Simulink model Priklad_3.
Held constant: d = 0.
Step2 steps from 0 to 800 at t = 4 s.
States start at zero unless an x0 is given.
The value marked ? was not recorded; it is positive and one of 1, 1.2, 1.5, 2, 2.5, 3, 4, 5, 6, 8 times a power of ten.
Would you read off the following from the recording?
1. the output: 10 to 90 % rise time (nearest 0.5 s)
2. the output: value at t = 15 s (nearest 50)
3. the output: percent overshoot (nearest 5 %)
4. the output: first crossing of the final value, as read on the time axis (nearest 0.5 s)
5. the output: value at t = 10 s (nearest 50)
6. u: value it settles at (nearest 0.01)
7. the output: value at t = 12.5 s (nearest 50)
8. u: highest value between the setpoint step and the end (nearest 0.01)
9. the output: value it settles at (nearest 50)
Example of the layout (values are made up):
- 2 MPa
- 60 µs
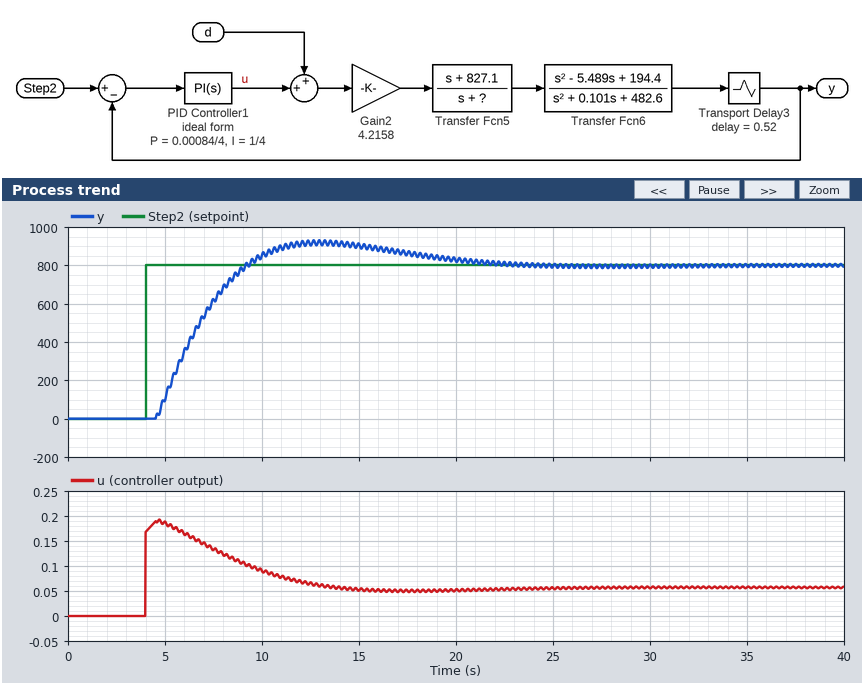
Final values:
- 3.5 s
- 900
- 15 %
- 9.0 s
- 850
- 0.06
- 900
- 0.19
- 800
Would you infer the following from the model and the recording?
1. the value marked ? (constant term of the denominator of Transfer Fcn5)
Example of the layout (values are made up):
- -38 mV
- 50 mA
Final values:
- 0.1
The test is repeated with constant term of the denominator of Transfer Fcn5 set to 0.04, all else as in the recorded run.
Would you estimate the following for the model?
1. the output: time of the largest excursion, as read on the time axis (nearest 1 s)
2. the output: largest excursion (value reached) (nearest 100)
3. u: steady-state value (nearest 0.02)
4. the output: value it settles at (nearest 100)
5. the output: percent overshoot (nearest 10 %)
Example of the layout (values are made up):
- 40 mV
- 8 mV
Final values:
- 12 s
- 1000
- 0.02
- 800
- 30 %
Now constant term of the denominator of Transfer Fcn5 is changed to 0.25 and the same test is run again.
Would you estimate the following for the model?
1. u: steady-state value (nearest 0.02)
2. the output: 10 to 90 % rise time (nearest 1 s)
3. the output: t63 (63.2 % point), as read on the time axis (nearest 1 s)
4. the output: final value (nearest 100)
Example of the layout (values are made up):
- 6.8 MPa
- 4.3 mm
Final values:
- 0.14
- 6 s
- 7 s
- 800
